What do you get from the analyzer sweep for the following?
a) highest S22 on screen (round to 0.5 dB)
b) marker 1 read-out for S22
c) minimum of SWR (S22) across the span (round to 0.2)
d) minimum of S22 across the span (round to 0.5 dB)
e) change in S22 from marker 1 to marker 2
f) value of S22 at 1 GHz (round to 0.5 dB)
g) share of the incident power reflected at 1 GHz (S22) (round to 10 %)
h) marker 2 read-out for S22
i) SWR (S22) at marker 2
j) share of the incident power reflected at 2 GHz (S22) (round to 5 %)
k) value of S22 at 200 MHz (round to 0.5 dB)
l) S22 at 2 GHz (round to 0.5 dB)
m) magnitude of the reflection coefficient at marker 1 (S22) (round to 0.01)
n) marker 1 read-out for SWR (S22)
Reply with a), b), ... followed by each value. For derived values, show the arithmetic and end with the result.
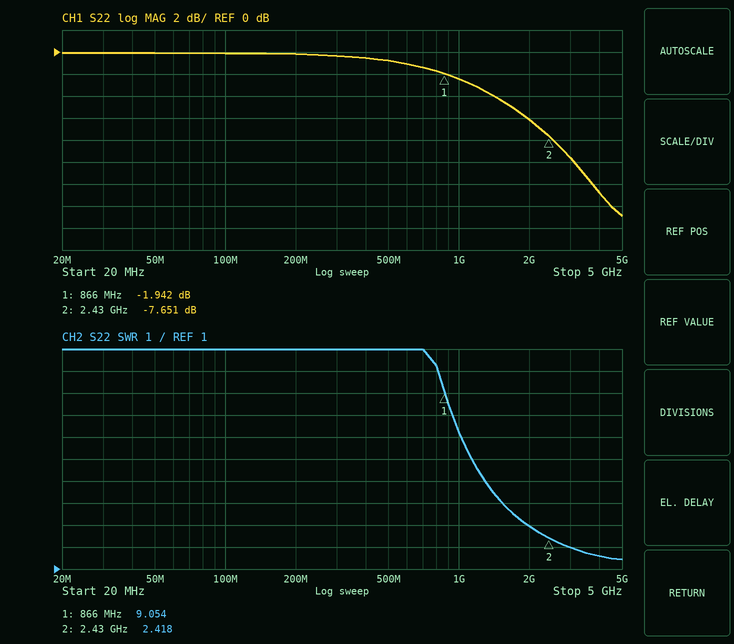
a) 0.0 dB
b) -1.942 dB
c) 1.4
d) -15.0 dB
e) -7.651 − (-1.942) = -5.709 dB
f) -2.5 dB
g) 10^(-2.5/10) ≈ 56.2 %, so 60 % to the nearest 10 %
h) -7.651 dB
i) 2.418
j) 10^(-6/10) ≈ 25 %
k) 0.0 dB
l) -6.0 dB
m) 10^(-1.942/20) ≈ 0.80
n) 9.054
